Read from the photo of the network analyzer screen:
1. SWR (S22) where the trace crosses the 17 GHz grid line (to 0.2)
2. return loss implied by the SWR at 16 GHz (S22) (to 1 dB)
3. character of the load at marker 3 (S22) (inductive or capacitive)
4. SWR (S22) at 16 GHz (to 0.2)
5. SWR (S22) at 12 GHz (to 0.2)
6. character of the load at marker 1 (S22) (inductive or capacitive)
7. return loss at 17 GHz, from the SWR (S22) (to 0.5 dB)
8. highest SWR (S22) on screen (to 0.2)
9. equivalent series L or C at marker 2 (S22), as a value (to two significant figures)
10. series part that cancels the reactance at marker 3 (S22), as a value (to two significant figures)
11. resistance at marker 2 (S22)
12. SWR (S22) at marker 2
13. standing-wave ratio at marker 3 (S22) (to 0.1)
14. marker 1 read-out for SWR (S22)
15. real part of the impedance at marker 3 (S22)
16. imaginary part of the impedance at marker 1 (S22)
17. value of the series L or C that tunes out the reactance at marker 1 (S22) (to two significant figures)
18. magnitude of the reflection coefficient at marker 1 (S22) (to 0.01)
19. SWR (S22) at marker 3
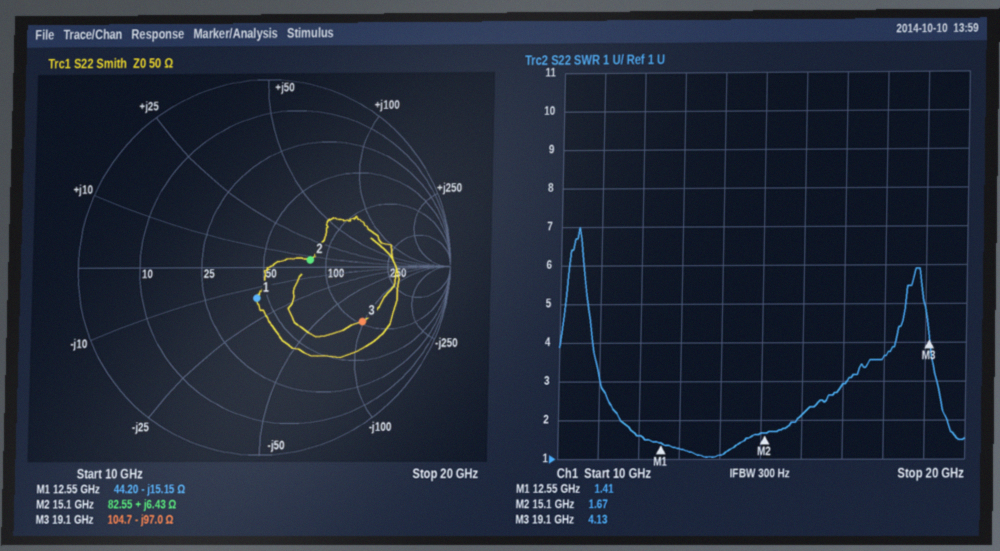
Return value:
3.0
9 dB
capacitive
2.2
1.6
capacitive
6.0 dB
7.0
68 pH
810 pH
82.55 Ω
1.67
4.1
1.41
104.7 Ω
-15.15 Ω
190 pH
0.17
4.13
